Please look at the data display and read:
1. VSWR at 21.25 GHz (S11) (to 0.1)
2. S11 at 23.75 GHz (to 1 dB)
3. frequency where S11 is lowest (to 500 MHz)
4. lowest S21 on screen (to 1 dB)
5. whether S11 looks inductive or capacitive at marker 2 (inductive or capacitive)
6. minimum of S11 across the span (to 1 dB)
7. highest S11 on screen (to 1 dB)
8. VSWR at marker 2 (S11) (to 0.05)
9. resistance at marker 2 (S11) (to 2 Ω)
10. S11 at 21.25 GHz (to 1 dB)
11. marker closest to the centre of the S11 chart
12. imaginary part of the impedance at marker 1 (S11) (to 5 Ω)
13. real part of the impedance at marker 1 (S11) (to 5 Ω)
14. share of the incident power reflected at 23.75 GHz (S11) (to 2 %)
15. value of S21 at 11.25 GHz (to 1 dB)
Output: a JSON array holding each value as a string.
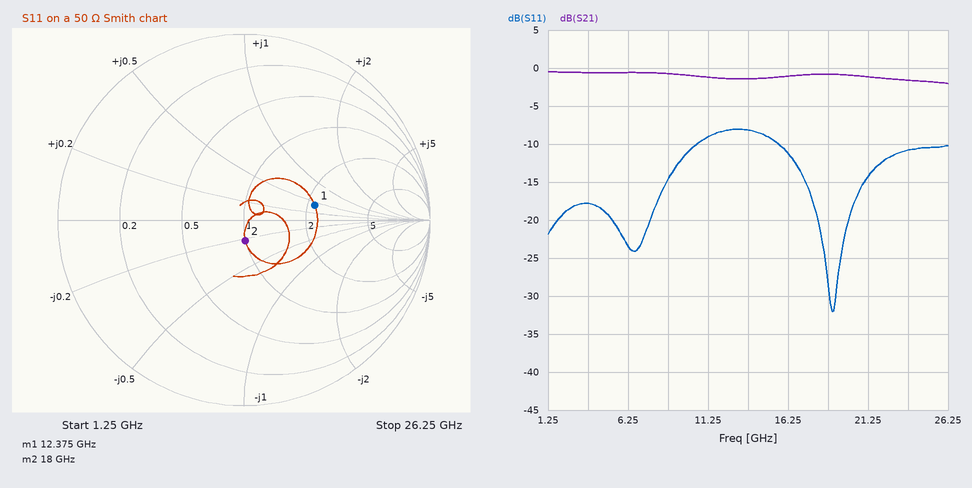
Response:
["1.5", "-11 dB", "19.0 GHz", "-2 dB", "capacitive", "-32 dB", "-8 dB", "1.25", "50 Ω", "-14 dB", "marker 2", "+20 Ω", "110 Ω", "8 %", "-1 dB"]
